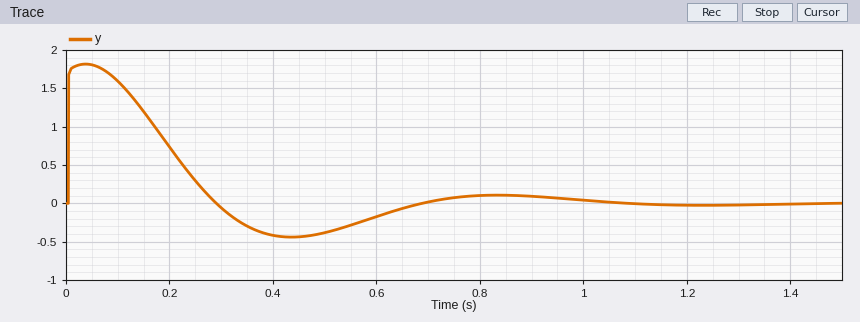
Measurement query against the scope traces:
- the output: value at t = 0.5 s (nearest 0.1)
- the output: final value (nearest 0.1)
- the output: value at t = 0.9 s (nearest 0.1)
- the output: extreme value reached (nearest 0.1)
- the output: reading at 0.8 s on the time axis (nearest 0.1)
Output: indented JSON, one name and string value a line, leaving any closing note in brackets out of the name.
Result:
{
  "the output: value at t = 0.5 s": "-0.4",
  "the output: final value": "0.0",
  "the output: value at t = 0.9 s": "0.1",
  "the output: extreme value reached": "1.8",
  "the output: reading at 0.8 s on the time axis": "0.1"
}
